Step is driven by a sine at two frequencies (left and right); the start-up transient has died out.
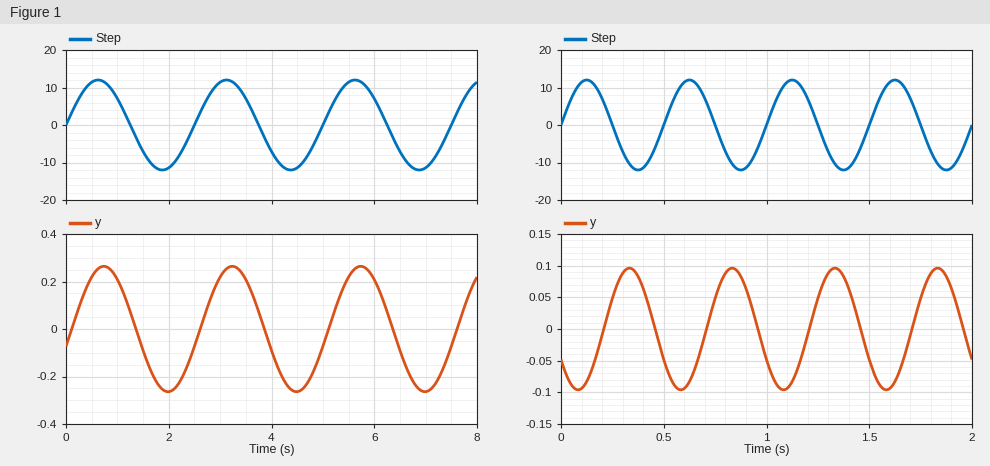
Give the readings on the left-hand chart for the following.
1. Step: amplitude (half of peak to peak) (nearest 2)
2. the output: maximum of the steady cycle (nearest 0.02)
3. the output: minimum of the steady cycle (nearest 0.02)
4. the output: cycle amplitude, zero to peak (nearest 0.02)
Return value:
12
0.26
-0.26
0.26
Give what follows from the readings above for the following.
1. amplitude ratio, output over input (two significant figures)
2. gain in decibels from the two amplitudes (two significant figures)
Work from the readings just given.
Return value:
0.022
-33 dB
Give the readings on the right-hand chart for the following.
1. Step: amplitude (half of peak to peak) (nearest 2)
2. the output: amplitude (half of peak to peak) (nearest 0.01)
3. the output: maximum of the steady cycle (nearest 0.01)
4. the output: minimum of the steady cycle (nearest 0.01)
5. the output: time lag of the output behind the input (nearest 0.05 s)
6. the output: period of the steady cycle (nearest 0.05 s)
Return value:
12
0.10
0.10
-0.10
0.20 s
0.50 s
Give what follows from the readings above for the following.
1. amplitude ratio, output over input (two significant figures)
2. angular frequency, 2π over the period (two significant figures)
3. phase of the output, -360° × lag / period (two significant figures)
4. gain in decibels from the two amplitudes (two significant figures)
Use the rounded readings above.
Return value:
0.0083
13 rad/s
-140°
-42 dB
